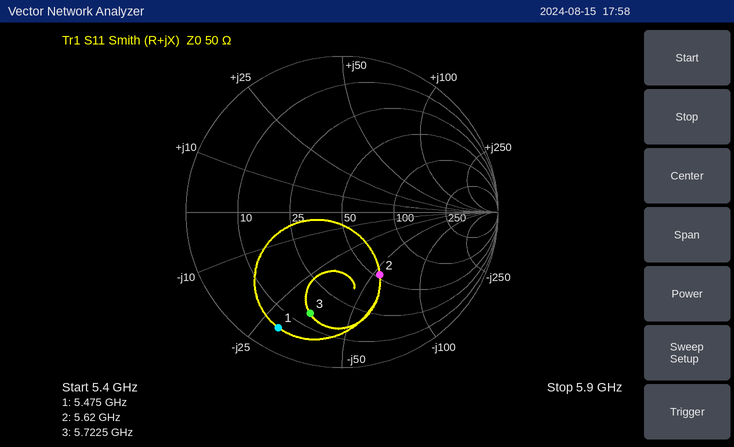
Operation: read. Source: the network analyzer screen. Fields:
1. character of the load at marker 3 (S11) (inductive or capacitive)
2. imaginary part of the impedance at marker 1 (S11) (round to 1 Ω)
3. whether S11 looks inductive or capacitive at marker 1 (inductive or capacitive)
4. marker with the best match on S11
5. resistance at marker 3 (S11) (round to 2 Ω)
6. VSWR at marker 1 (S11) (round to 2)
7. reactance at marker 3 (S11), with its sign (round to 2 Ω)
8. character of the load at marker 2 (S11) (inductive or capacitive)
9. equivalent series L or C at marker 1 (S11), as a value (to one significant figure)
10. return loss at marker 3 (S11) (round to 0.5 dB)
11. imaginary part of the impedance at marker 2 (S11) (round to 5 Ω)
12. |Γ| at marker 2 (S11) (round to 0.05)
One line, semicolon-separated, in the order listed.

capacitive; -29 Ω; capacitive; marker 2; 14 Ω; 12; -34 Ω; capacitive; 1.0 pF; 3.5 dB; -55 Ω; 0.45
